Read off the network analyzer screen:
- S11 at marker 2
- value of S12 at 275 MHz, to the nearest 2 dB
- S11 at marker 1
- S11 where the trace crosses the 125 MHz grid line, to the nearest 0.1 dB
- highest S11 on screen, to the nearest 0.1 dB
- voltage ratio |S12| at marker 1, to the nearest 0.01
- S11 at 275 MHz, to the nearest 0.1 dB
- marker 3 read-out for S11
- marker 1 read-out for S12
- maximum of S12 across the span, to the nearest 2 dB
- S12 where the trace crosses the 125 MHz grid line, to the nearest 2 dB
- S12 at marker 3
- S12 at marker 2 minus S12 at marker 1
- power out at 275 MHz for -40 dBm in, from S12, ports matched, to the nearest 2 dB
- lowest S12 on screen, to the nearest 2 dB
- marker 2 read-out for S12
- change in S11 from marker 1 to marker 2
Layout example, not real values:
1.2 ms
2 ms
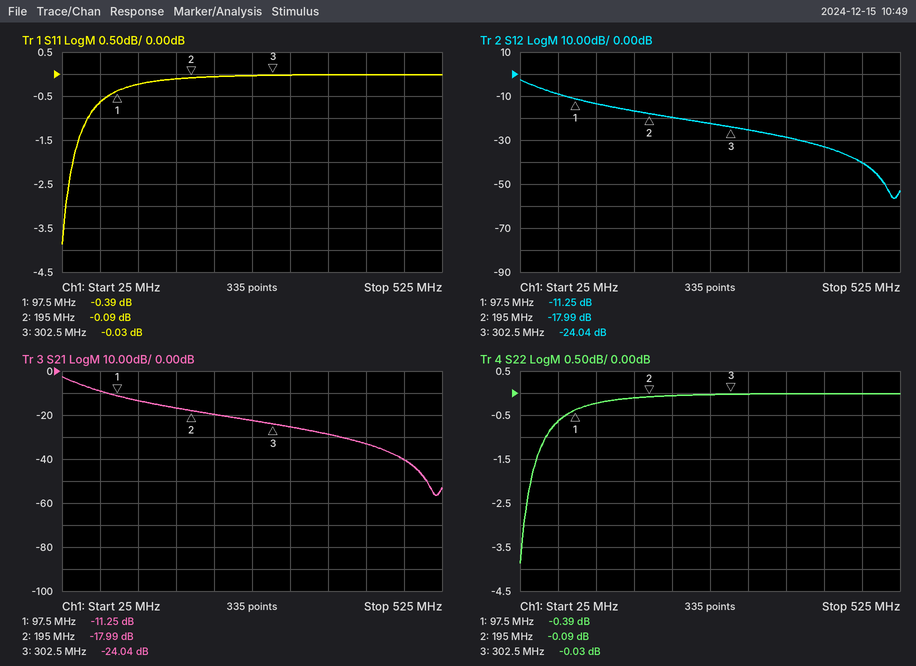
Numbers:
-0.09 dB
-22 dB
-0.39 dB
-0.2 dB
0.0 dB
0.27
0.0 dB
-0.03 dB
-11.25 dB
-2 dB
-14 dB
-24.04 dB
-6.74 dB
-62 dBm
-56 dB
-17.99 dB
0.30 dB
